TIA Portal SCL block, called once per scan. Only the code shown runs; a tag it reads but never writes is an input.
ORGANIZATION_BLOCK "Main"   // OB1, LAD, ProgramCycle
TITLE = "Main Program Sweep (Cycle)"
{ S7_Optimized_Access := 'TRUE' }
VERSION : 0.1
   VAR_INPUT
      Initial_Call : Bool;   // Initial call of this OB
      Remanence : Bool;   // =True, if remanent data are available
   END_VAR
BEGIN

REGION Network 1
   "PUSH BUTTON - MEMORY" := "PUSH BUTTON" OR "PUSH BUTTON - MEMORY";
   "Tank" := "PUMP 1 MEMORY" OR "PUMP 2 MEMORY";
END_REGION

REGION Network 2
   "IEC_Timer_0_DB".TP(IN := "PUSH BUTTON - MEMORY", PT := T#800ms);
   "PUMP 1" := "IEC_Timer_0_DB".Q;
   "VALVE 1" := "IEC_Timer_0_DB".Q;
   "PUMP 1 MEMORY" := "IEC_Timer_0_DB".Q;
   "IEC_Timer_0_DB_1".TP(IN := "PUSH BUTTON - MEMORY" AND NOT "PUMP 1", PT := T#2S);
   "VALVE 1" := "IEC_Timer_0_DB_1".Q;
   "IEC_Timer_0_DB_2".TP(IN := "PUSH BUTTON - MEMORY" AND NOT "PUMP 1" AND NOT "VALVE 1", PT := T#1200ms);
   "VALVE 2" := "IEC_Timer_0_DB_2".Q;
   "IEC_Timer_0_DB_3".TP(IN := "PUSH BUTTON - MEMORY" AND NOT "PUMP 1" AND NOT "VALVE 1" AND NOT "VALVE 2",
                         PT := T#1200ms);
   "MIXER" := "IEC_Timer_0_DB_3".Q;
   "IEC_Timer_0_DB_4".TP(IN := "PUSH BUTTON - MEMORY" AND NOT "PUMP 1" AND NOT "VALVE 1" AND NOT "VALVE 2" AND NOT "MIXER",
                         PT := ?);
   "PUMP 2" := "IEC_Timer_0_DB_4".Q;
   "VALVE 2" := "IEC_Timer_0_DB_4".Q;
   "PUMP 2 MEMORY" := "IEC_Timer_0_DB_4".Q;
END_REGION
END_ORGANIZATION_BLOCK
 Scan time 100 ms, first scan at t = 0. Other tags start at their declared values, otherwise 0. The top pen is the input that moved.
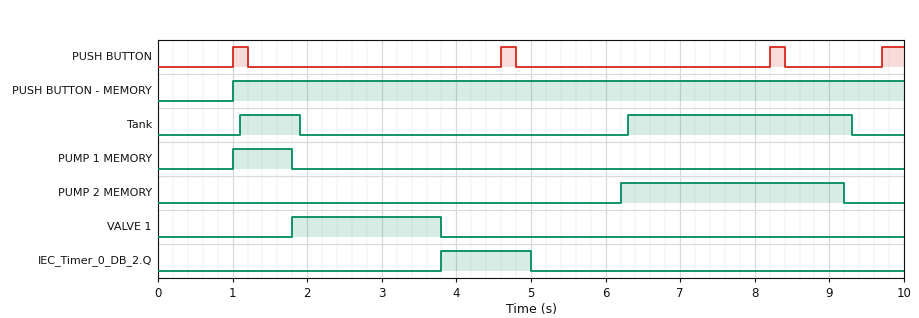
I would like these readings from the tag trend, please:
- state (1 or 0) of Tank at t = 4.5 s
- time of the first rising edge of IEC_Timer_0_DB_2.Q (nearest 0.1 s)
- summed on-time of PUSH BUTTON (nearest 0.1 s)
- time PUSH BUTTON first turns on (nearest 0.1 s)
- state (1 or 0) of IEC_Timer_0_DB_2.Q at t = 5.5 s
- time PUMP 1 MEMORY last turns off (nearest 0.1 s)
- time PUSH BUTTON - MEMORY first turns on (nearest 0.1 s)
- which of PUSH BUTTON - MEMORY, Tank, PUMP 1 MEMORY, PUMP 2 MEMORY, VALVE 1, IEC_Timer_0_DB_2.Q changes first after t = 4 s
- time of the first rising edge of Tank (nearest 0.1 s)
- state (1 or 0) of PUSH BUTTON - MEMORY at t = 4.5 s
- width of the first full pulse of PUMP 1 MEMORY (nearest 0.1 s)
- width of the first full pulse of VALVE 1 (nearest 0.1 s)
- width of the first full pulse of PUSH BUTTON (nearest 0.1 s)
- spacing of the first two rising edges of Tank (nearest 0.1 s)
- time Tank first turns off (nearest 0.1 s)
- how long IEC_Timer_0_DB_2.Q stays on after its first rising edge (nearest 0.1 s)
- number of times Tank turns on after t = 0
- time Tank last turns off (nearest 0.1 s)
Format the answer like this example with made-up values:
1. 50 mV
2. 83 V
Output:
1. 0
2. 3.8 s
3. 0.9 s
4. 1.0 s
5. 0
6. 1.8 s
7. 1.0 s
8. IEC_Timer_0_DB_2.Q
9. 1.1 s
10. 1
11. 0.8 s
12. 2.0 s
13. 0.2 s
14. 5.2 s
15. 1.9 s
16. 1.2 s
17. 2
18. 9.3 s
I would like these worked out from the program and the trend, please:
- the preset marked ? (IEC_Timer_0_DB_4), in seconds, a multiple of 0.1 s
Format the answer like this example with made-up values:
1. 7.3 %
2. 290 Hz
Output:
1. 3.0 s
